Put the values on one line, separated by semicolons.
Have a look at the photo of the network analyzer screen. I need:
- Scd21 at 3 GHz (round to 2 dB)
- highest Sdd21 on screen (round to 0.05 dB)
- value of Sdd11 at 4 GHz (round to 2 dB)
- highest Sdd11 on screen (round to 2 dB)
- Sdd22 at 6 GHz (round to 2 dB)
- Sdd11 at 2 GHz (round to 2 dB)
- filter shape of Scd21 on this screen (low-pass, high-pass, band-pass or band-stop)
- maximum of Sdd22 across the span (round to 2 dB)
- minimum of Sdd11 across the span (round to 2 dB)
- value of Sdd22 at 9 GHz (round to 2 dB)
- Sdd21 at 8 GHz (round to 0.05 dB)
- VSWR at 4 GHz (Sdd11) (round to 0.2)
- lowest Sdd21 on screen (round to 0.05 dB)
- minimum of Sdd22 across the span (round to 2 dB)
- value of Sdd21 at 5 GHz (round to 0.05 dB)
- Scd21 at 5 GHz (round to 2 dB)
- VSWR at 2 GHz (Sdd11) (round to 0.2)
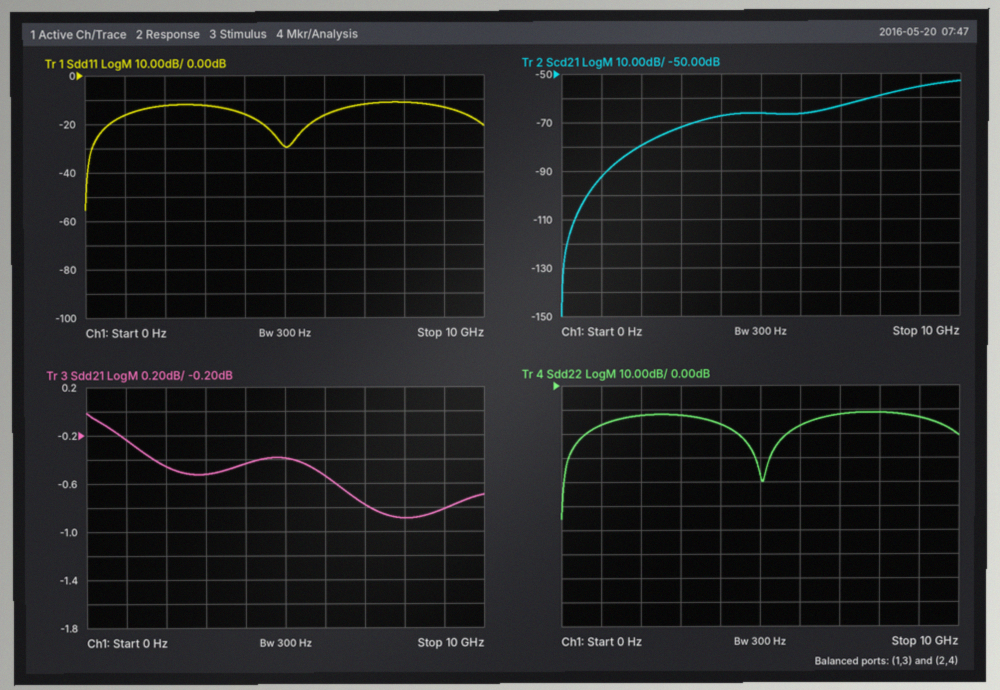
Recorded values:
-72 dB; 0.00 dB; -16 dB; -12 dB; -16 dB; -12 dB; high-pass; -12 dB; -56 dB; -14 dB; -0.90 dB; 1.4; -0.90 dB; -56 dB; -0.40 dB; -66 dB; 1.6
